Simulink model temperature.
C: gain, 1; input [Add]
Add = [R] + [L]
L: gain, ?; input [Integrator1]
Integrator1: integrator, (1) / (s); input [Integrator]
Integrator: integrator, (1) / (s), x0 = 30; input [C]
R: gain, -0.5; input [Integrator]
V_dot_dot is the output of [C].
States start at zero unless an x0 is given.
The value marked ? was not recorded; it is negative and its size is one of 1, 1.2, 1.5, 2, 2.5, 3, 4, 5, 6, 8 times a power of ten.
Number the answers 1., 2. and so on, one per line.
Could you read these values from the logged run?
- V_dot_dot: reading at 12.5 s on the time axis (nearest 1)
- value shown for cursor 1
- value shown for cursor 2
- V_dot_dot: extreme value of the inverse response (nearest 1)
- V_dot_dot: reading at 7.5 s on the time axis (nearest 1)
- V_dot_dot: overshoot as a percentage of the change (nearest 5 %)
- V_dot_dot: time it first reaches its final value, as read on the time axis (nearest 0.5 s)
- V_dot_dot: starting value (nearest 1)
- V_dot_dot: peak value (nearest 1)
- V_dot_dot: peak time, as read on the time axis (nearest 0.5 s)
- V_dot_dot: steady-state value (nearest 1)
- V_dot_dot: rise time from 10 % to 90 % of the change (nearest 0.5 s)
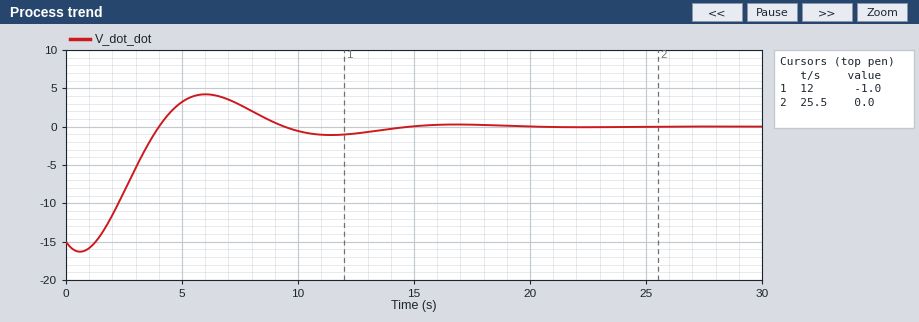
1. -1
2. -1.0
3. 0.0
4. -16
5. 3
6. 30 %
7. 4.0 s
8. -15
9. 4
10. 6.0 s
11. 0
12. 2.0 s
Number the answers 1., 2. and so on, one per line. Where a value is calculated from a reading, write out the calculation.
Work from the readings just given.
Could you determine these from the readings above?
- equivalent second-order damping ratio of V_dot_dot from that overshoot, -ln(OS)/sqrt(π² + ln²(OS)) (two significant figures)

1. ln(0.3) = -1.204; 1.204 / sqrt(9.870 + 1.450) = 0.36
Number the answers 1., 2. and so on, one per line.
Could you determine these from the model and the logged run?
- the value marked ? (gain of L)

1. -0.4
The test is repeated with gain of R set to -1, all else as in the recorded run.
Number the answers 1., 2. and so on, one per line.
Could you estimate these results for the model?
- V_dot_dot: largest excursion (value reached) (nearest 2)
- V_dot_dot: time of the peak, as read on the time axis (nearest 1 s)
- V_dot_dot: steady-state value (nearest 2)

1. 2
2. 5 s
3. 0
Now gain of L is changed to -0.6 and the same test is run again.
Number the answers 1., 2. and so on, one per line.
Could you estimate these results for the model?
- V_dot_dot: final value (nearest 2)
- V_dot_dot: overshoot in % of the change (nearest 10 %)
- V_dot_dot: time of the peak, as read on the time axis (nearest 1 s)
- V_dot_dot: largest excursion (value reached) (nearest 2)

1. 0
2. 40 %
3. 5 s
4. 6
